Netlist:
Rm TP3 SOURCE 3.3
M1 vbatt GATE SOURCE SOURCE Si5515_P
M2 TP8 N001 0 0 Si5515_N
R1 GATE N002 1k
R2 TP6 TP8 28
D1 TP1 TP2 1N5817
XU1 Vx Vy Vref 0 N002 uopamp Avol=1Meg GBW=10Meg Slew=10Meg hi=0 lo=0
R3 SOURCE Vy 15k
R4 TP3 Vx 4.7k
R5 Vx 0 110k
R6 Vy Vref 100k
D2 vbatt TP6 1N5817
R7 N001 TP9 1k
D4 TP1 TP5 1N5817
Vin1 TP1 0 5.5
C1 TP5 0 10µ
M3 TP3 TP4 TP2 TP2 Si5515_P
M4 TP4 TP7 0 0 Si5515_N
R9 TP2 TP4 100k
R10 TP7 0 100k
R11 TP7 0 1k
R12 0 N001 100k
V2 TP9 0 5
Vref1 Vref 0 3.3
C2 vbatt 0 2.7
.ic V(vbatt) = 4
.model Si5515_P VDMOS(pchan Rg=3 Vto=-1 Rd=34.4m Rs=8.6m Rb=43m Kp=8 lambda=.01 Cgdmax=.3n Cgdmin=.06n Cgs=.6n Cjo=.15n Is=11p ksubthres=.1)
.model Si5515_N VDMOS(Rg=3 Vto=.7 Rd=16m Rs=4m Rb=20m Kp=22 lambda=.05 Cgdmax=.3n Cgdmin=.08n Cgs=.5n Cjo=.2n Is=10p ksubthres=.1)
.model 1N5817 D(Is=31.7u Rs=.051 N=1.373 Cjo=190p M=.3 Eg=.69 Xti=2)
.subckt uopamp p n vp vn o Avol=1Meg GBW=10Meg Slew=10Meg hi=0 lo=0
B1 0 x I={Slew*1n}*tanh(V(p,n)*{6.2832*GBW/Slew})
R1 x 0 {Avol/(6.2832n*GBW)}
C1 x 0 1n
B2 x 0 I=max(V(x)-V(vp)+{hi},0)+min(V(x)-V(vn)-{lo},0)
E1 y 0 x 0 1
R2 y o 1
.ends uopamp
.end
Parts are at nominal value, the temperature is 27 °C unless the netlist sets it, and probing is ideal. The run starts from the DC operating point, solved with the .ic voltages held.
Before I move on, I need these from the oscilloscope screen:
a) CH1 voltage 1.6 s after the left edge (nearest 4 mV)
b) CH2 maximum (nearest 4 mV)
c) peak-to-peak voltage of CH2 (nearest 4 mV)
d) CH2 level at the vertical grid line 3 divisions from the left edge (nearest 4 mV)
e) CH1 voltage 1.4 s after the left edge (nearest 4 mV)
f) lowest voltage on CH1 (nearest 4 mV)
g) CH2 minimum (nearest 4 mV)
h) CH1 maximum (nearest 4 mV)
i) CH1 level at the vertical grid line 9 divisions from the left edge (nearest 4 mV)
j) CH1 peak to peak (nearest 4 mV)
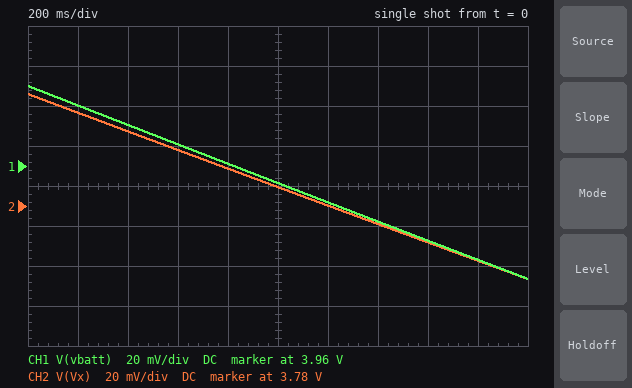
3.924 V
3.836 V
92 mV
3.808 V
3.932 V
3.904 V
3.744 V
4.000 V
3.912 V
96 mV
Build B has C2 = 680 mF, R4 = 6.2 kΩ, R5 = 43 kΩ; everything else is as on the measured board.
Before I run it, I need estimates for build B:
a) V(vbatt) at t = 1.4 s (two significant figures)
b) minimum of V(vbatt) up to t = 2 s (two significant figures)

3.7 V
3.6 V
